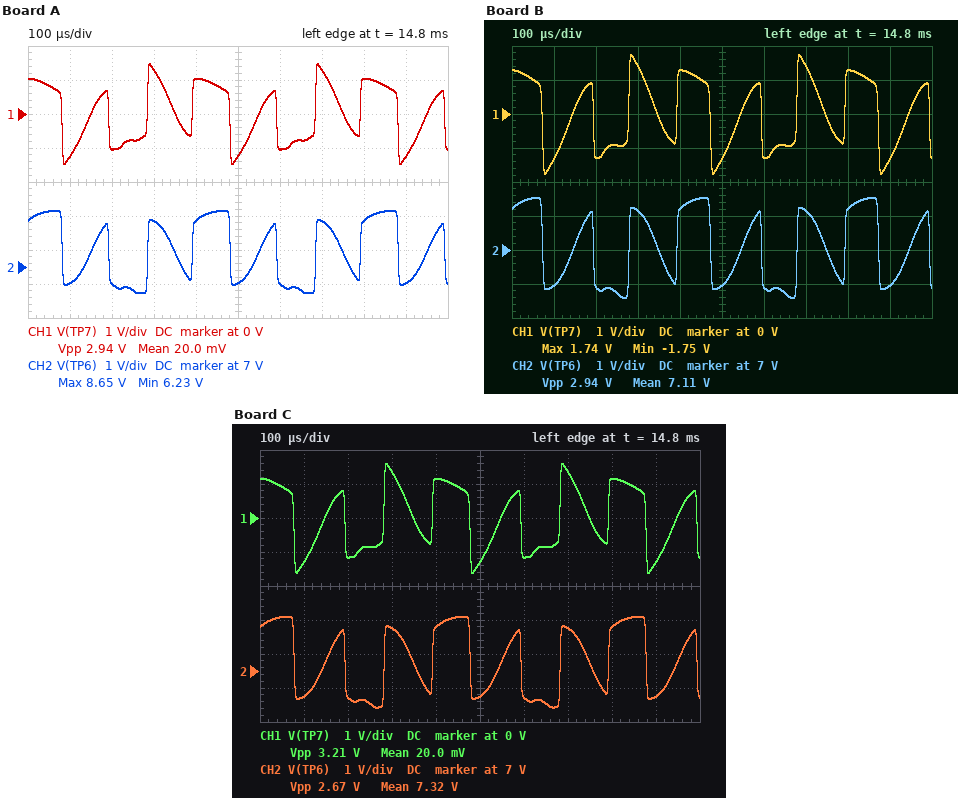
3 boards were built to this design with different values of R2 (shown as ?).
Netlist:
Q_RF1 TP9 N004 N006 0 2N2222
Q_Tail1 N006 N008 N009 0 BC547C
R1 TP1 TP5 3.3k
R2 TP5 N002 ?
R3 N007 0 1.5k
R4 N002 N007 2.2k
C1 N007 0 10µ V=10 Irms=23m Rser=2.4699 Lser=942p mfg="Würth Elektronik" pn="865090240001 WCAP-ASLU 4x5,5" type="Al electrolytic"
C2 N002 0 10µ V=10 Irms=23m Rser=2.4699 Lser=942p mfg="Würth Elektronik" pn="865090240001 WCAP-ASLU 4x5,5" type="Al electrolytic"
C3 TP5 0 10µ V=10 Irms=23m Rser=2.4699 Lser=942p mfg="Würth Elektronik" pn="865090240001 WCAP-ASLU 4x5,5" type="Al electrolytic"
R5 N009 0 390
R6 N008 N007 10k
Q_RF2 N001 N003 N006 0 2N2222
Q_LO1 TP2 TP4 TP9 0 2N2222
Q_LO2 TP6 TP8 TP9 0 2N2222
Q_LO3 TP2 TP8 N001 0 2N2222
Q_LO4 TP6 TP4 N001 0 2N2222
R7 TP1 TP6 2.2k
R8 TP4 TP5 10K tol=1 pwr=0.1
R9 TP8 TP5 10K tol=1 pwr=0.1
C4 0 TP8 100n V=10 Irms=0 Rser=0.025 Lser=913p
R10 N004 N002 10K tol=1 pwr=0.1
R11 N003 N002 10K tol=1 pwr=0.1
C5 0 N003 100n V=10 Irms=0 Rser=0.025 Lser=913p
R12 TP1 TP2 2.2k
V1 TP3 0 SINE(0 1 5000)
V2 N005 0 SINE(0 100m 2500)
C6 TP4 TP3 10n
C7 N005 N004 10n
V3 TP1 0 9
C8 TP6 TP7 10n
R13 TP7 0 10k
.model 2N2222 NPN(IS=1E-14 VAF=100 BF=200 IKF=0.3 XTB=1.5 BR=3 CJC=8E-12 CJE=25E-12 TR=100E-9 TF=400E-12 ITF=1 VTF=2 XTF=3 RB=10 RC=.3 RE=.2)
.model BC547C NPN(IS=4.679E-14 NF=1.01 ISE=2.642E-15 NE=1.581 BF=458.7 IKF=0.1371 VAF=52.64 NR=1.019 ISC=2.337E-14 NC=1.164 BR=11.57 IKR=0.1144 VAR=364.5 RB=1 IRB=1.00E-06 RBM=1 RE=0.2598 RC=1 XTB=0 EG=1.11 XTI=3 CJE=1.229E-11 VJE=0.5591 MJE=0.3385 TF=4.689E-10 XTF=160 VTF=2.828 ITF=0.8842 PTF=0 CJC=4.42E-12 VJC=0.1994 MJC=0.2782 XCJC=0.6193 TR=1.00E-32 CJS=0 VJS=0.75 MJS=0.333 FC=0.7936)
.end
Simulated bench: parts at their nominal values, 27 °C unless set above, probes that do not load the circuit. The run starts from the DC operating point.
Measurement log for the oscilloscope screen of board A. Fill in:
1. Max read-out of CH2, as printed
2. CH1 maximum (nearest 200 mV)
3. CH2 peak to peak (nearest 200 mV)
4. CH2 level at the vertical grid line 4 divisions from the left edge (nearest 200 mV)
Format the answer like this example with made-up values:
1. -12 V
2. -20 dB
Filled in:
1. 8.65 V
2. 1.4 V
3. 2.4 V
4. 8.4 V
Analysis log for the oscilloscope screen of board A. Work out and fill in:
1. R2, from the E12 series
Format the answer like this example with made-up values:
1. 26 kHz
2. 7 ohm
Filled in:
1. 3.9 kΩ
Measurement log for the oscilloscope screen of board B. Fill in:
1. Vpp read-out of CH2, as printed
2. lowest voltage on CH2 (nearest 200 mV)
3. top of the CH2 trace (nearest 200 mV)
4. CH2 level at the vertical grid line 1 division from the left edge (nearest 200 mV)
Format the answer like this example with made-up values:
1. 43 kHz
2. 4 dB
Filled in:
1. 2.94 V
2. 5.6 V
3. 8.6 V
4. 6.0 V
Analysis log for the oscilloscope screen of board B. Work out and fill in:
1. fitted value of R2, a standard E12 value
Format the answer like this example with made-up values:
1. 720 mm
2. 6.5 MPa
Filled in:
1. 2.7 kΩ
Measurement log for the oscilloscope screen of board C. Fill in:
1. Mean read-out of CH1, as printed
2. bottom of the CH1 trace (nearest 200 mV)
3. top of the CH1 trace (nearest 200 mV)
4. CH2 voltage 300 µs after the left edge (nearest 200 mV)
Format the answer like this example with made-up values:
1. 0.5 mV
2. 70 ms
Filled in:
1. 20.0 mV
2. -1.6 V
3. 1.6 V
4. 8.2 V
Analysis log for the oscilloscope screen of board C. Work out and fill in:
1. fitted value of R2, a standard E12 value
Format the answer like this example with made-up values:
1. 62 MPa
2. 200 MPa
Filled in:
1. 3.3 kΩ
